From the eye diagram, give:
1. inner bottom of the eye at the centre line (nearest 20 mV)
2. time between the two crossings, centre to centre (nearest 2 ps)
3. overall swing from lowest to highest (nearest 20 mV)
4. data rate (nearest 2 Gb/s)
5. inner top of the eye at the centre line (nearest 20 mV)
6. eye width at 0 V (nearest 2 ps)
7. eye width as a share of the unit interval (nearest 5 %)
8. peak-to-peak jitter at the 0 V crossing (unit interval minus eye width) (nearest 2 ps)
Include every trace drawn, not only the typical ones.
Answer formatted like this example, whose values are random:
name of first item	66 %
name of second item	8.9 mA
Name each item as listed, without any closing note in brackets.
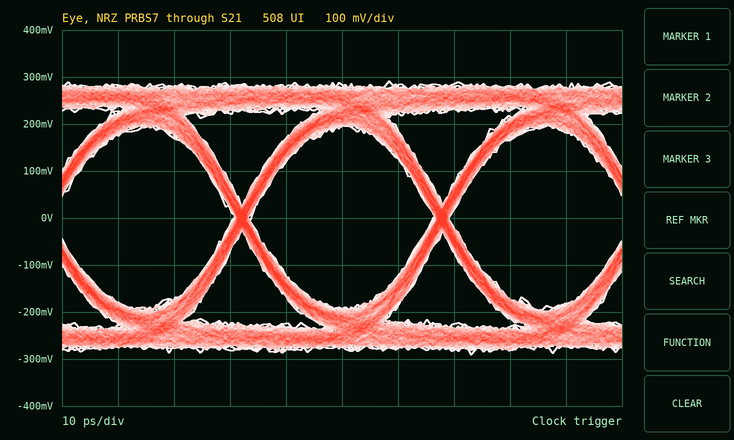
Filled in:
inner bottom of the eye at the centre line	-200 mV
time between the two crossings, centre to centre	36 ps
overall swing from lowest to highest	580 mV
data rate	28 Gb/s
inner top of the eye at the centre line	200 mV
eye width at 0 V	32 ps
eye width as a share of the unit interval	90 %
peak-to-peak jitter at the 0 V crossing (unit interval minus eye width)	4 ps
